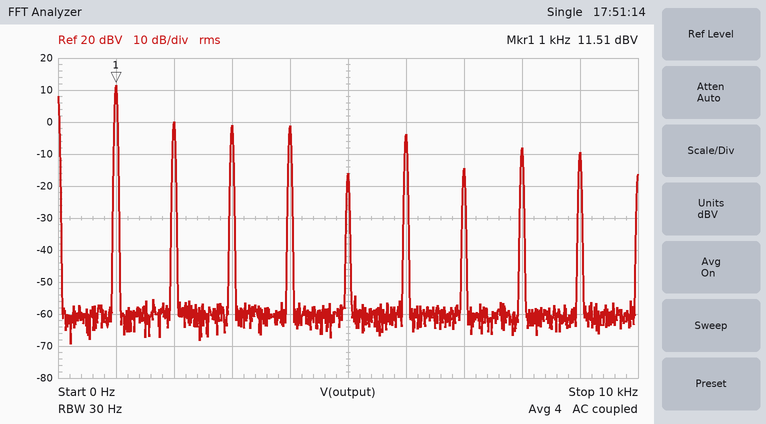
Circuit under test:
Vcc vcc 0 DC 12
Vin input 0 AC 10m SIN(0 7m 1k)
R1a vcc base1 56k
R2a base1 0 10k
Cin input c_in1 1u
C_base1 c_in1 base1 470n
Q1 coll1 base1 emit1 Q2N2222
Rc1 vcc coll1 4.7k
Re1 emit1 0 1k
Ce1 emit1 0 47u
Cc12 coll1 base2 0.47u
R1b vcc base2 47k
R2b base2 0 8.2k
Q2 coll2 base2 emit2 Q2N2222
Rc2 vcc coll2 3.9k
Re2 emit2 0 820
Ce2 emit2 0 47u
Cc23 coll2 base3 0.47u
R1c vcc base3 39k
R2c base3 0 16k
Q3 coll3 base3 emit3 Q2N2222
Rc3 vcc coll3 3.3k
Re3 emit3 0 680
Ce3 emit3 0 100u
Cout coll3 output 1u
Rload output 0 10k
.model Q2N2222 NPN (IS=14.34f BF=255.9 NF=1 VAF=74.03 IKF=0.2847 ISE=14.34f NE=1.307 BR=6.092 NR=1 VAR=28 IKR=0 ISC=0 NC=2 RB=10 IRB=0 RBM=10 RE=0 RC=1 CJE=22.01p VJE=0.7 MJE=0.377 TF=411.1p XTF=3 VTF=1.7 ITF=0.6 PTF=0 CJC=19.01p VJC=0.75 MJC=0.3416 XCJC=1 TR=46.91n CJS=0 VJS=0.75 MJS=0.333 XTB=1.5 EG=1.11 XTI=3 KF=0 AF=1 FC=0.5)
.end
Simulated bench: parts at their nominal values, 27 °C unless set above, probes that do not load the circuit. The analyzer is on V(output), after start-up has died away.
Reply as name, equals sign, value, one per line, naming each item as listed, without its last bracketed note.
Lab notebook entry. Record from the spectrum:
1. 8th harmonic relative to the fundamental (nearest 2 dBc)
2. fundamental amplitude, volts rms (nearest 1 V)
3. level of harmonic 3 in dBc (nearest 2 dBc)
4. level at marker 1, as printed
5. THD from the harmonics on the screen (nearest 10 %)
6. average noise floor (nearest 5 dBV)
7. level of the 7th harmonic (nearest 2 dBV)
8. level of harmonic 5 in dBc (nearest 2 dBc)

8th harmonic relative to the fundamental = -20 dBc
fundamental amplitude, volts rms = 4 V
level of harmonic 3 in dBc = -12 dBc
level at marker 1, as printed = 11.51 dBV
THD from the harmonics on the screen = 50 %
average noise floor = -60 dBV
level of the 7th harmonic = -14 dBV
level of harmonic 5 in dBc = -28 dBc
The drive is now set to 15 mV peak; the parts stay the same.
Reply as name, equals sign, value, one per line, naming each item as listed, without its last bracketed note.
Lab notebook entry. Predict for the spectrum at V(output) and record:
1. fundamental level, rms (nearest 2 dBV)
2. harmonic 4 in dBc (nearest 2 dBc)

fundamental level, rms = 12 dBV
harmonic 4 in dBc = -14 dBc
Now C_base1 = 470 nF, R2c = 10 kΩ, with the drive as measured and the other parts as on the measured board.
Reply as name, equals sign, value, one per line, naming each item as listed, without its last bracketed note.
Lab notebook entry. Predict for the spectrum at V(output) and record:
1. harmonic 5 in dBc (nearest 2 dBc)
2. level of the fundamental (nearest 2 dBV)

harmonic 5 in dBc = -36 dBc
level of the fundamental = 12 dBV
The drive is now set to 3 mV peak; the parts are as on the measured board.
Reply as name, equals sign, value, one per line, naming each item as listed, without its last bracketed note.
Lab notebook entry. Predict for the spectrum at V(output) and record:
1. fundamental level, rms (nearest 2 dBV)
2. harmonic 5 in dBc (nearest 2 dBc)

fundamental level, rms = 12 dBV
harmonic 5 in dBc = -24 dBc
